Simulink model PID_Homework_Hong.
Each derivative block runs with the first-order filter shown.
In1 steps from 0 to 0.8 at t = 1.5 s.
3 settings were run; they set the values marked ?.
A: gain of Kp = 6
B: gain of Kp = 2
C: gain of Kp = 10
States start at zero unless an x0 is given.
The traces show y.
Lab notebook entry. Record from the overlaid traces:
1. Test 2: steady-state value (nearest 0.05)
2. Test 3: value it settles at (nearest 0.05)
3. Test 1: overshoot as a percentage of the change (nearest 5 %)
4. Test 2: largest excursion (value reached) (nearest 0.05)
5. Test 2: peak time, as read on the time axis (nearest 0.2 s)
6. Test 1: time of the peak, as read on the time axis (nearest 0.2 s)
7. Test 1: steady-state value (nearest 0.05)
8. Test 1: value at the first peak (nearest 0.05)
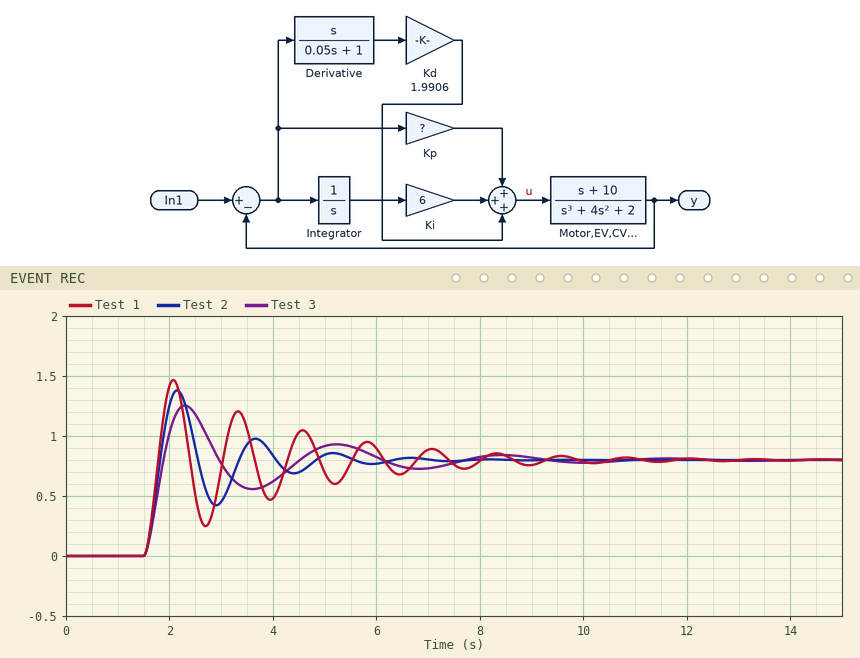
0.80
0.80
85 %
1.40
2.2 s
2.0 s
0.80
1.45
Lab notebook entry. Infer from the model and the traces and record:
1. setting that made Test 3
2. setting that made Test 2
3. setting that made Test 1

B
A
C
